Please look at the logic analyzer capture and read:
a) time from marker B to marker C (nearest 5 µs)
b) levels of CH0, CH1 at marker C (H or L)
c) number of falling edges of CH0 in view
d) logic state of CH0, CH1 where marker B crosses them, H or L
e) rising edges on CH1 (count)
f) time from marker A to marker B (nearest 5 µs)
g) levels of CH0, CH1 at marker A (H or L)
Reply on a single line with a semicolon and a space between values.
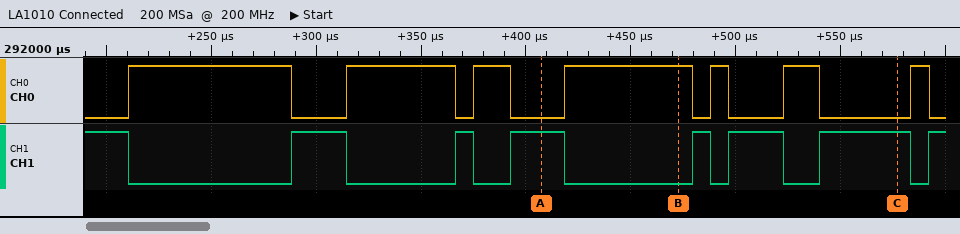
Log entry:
105 µs; CH0=L, CH1=H; 7; CH0=H, CH1=L; 7; 65 µs; CH0=L, CH1=H
